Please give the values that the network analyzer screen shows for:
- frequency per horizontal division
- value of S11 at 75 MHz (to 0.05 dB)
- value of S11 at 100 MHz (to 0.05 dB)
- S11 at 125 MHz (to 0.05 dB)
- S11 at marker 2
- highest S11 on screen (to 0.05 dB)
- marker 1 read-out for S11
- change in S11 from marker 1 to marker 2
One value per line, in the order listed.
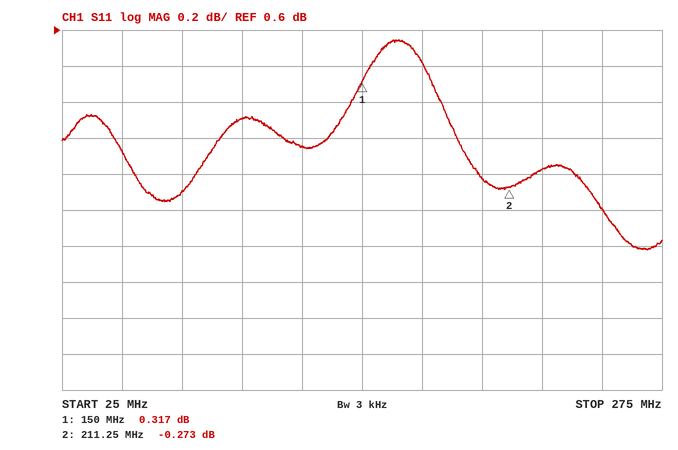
25 MHz
-0.30 dB
0.10 dB
-0.05 dB
-0.273 dB
0.55 dB
0.317 dB
-0.590 dB
